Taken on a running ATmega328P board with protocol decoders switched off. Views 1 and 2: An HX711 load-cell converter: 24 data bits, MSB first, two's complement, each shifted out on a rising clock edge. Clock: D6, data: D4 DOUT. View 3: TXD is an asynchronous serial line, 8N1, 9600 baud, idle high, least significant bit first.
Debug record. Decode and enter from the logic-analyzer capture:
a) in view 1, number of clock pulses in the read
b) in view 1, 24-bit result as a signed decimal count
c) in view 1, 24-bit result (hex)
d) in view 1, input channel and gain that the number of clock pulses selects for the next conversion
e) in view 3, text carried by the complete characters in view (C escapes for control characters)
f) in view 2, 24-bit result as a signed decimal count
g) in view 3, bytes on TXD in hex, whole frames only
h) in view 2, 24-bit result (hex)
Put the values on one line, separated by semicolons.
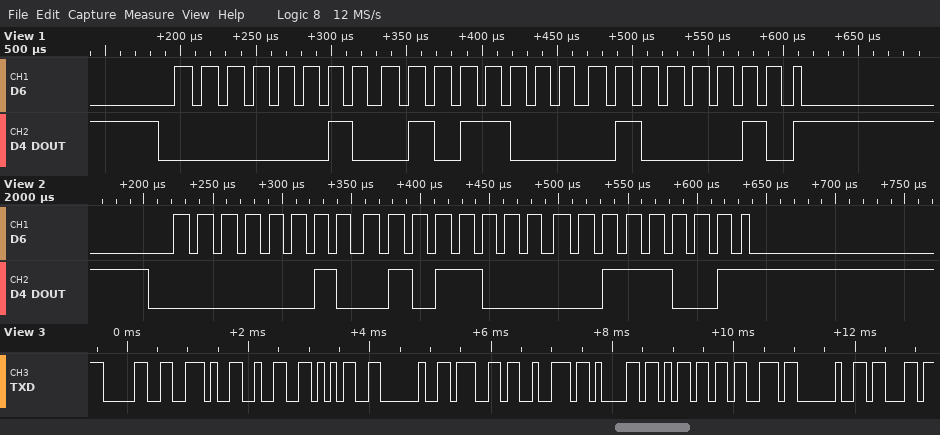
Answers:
25; 153666; 0x025842; channel A, gain 128; "0.25 grams c"; 153657; 30 2E 32 35 20 67 72 61 6D 73 20 63; 0x025839
